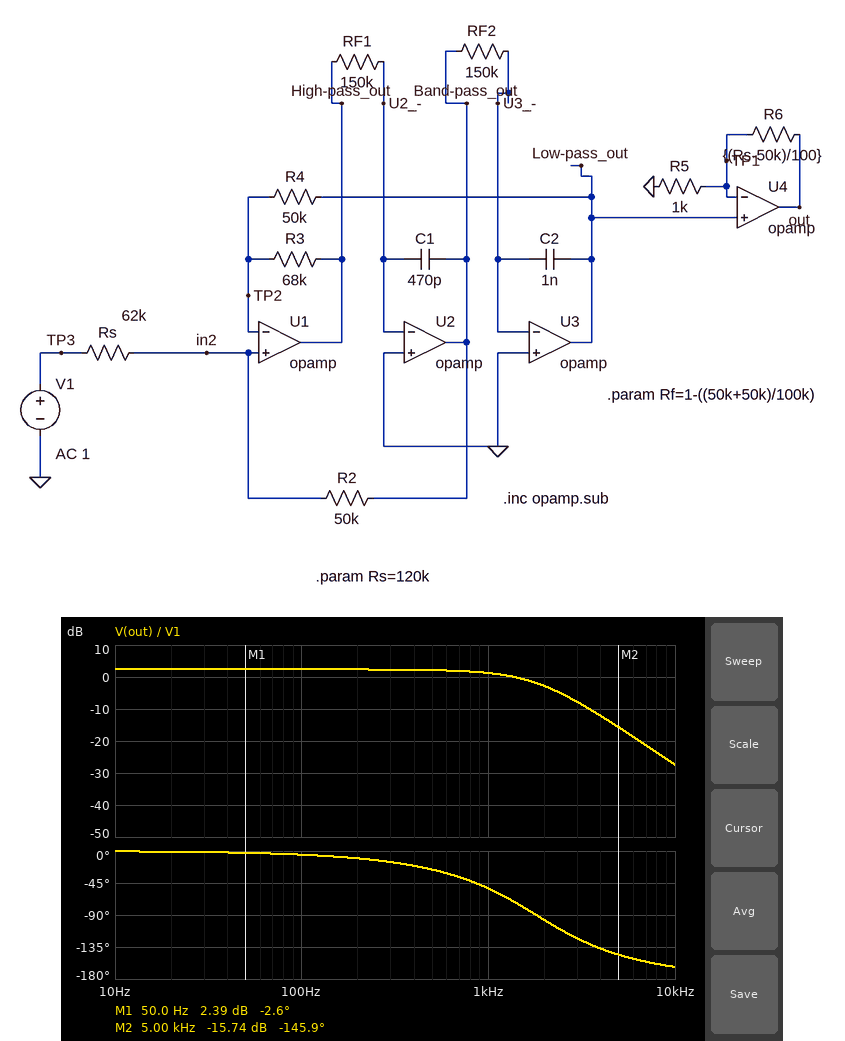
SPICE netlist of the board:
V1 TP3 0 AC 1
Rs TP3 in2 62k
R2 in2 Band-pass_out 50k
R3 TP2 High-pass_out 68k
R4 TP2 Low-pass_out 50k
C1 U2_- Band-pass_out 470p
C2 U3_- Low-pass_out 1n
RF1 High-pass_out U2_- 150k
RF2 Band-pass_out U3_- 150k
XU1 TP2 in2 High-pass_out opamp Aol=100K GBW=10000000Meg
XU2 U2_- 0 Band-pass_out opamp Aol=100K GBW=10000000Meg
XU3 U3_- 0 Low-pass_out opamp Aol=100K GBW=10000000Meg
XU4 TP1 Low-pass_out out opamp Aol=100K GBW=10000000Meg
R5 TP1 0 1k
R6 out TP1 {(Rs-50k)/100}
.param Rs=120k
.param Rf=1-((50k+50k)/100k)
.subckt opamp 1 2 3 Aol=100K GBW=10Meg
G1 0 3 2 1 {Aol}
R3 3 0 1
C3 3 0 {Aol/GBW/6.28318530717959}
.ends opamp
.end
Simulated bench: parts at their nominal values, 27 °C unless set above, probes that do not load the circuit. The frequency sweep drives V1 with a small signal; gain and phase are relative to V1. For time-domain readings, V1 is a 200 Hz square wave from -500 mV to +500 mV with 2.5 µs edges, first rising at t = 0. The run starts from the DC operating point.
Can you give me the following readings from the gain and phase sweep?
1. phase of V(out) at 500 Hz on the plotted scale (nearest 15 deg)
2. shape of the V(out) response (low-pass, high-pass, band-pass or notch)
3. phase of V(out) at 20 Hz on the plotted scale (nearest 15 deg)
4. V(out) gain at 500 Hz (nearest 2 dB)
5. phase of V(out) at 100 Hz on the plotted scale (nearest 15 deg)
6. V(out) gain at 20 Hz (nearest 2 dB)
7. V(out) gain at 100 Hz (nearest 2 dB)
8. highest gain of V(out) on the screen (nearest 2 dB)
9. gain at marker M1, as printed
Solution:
-30 deg
low-pass
0 deg
2 dB
0 deg
2 dB
2 dB
2 dB
2.39 dB
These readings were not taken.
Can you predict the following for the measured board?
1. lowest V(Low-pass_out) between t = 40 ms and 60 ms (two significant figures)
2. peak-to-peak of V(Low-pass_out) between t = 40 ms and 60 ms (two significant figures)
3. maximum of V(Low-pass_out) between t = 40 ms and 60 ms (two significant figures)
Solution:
-400 mV
790 mV
400 mV
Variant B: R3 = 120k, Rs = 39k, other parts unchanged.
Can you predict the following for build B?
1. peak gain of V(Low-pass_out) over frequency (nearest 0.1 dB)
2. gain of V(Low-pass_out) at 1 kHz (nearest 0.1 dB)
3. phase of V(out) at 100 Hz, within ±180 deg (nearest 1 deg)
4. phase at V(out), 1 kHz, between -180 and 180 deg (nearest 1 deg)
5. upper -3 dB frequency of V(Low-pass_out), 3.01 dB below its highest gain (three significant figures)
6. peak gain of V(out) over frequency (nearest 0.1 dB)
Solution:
-2.0 dB
-2.1 dB
-3 deg
-35 deg
2.42 kHz
2.6 dB
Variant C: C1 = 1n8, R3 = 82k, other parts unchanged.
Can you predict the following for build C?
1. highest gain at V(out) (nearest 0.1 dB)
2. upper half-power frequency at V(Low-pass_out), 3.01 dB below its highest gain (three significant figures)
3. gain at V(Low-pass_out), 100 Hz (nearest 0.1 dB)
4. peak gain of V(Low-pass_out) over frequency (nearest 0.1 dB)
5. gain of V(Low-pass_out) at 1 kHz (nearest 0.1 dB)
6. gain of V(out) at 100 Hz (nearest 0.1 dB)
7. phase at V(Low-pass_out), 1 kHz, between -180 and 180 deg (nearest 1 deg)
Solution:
4.0 dB
1.20 kHz
-2.8 dB
-0.6 dB
-1.4 dB
1.8 dB
-88 deg
